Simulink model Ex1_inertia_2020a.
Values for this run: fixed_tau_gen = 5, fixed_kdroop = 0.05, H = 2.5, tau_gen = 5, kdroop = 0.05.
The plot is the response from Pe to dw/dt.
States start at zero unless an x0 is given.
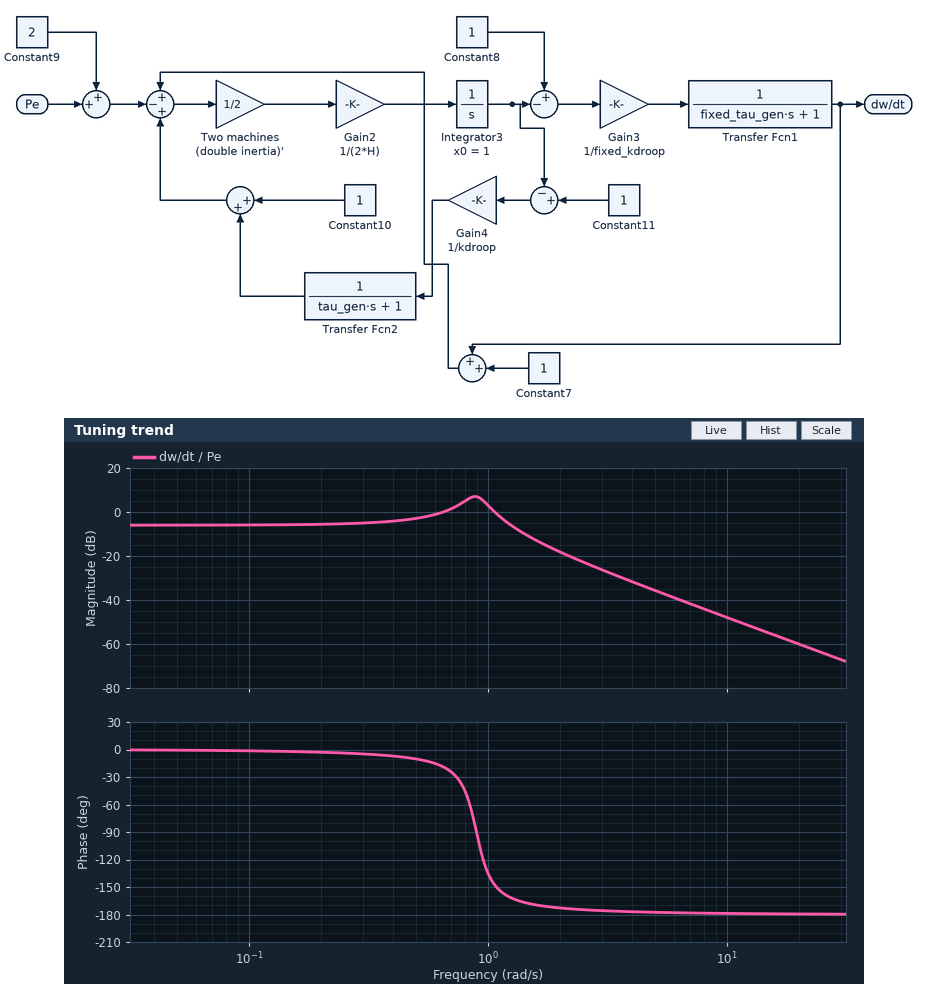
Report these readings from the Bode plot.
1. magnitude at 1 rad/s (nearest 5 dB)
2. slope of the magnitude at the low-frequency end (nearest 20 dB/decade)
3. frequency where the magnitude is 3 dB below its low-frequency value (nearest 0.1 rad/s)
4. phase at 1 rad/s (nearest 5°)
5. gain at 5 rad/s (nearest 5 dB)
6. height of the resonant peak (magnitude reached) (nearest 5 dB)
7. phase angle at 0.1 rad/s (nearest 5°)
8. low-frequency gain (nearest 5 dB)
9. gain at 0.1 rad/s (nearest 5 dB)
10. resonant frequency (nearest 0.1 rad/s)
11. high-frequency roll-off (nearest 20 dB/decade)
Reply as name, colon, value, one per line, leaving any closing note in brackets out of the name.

magnitude at 1 rad/s: 5 dB
slope of the magnitude at the low-frequency end: 0 dB/decade
frequency where the magnitude is 3 dB below its low-frequency value: 1.4 rad/s
phase at 1 rad/s: -135°
gain at 5 rad/s: -35 dB
height of the resonant peak (magnitude reached): 5 dB
phase angle at 0.1 rad/s: 0°
low-frequency gain: -5 dB
gain at 0.1 rad/s: -5 dB
resonant frequency: 0.9 rad/s
high-frequency roll-off: -40 dB/decade
